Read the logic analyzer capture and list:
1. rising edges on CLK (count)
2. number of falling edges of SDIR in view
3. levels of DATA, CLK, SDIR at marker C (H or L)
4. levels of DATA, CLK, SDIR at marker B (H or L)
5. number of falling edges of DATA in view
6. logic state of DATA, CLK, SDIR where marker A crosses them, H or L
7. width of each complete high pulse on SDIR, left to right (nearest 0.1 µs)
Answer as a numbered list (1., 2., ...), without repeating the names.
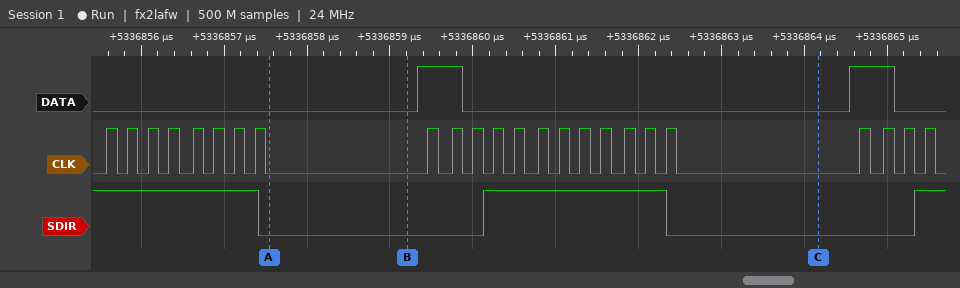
1. 24
2. 2
3. DATA=L, CLK=L, SDIR=L
4. DATA=L, CLK=L, SDIR=L
5. 2
6. DATA=L, CLK=L, SDIR=L
7. 2.2 µs
